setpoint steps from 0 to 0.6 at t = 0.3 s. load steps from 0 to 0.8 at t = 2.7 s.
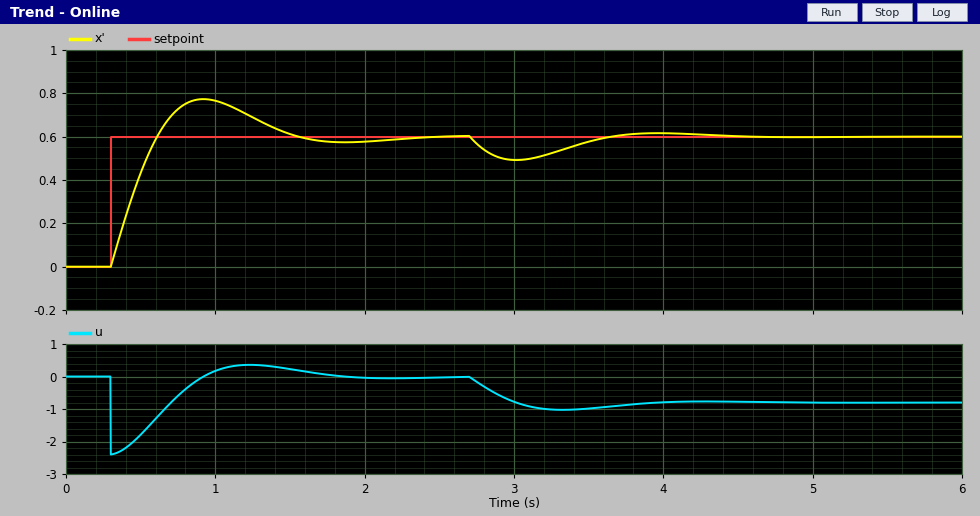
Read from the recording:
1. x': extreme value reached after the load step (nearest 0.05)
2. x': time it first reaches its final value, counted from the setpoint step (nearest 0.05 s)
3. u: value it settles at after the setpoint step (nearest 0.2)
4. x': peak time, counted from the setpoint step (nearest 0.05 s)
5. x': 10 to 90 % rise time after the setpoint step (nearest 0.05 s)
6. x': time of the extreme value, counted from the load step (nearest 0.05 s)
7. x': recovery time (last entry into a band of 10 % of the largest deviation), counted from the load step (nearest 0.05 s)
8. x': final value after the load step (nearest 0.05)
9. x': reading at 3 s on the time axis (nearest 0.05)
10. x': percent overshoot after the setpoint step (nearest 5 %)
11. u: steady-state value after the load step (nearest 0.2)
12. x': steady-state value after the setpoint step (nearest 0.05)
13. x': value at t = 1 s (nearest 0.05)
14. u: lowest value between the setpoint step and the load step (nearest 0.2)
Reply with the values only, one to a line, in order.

0.50
0.30 s
0.0
0.60 s
0.25 s
0.30 s
1.50 s
0.60
0.50
30 %
-0.8
0.60
0.75
-2.4
